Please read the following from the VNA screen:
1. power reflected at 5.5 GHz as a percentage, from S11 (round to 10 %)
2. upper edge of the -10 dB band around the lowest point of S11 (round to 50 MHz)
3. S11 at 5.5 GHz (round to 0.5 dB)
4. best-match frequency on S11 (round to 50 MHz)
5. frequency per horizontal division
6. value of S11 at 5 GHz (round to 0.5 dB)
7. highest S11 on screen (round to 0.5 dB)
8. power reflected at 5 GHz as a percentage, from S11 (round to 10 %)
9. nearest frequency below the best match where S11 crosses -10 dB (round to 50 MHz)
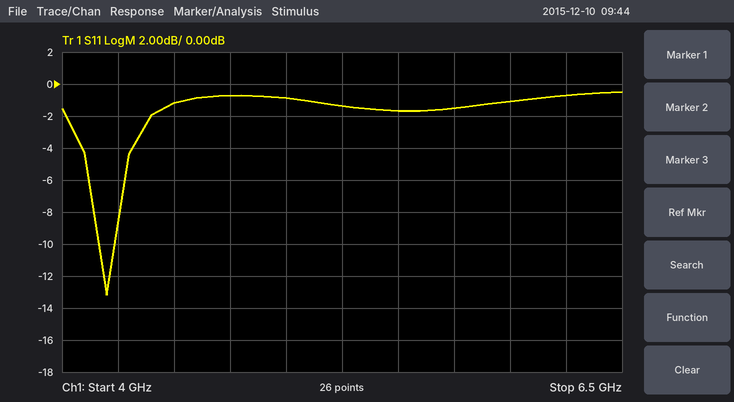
70 %
4.25 GHz
-1.5 dB
4.20 GHz
250 MHz
-1.0 dB
-0.5 dB
80 %
4.15 GHz
